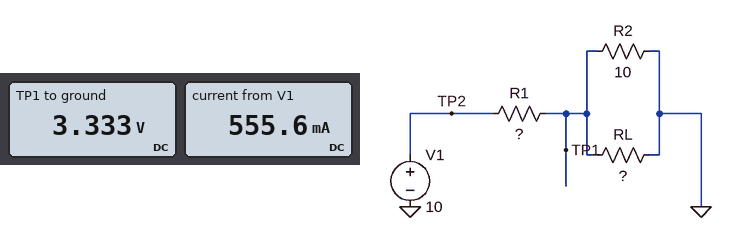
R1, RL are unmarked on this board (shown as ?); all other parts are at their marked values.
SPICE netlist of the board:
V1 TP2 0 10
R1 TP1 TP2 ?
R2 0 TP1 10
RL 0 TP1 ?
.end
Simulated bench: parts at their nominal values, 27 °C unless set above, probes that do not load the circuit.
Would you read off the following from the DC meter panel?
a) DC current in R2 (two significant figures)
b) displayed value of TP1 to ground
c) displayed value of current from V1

330 mA
3.333 V
555.6 mA
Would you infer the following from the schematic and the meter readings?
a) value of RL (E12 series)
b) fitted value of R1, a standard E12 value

15 Ω
12 Ω
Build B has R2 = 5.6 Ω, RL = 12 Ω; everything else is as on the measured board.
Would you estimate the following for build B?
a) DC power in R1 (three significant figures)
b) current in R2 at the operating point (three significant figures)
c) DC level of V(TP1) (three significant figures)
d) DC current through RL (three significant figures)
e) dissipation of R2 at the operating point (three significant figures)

4.80 W
431 mA
2.41 V
201 mA
1.04 W
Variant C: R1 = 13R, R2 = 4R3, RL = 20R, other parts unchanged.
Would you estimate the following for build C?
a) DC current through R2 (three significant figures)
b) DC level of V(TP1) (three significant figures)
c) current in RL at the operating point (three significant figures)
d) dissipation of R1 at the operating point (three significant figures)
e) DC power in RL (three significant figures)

498 mA
2.14 V
107 mA
4.75 W
229 mW
